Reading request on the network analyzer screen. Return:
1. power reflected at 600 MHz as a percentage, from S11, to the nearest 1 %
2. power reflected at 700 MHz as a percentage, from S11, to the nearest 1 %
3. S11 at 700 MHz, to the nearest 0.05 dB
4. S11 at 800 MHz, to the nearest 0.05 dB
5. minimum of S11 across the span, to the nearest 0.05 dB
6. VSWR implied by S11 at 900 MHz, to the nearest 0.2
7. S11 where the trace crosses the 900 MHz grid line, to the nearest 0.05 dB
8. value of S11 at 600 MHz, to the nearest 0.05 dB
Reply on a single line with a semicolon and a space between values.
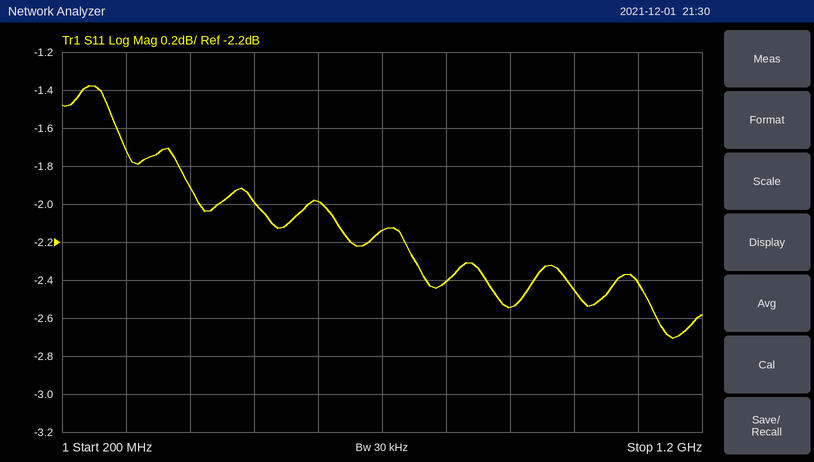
63 %; 61 %; -2.15 dB; -2.40 dB; -2.70 dB; 6.8; -2.55 dB; -2.00 dB
